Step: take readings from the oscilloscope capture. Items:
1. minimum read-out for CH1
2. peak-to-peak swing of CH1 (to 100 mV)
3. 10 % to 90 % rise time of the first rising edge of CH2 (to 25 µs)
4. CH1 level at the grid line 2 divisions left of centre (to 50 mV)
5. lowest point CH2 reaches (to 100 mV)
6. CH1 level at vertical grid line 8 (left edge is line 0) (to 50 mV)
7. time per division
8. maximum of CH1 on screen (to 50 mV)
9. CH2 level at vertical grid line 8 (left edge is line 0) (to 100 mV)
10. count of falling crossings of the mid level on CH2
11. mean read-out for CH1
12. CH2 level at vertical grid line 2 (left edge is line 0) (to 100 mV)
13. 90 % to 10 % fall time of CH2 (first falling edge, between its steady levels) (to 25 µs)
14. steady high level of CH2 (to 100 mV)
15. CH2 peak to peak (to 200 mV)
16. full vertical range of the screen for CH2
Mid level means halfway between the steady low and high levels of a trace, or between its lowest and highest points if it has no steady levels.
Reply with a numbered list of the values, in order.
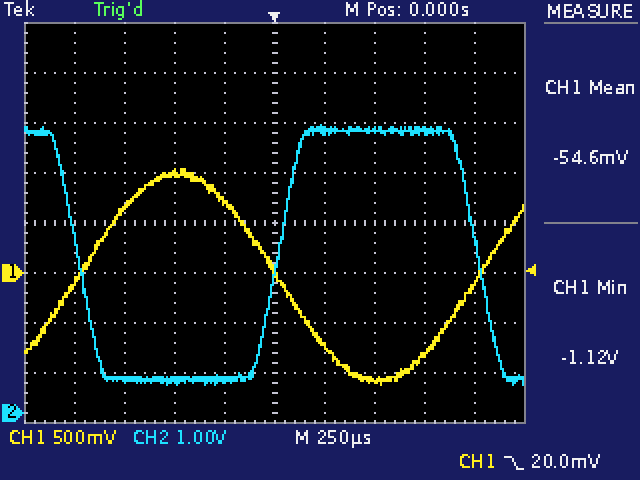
1. -1.12 V
2. 2.20 V
3. 200 µs
4. 1.00 V
5. 600 mV
6. -800 mV
7. 250 µs
8. 1.05 V
9. 5.6 V
10. 2
11. -54.6 mV
12. 700 mV
13. 200 µs
14. 5.6 V
15. 5.2 V
16. 8 V
